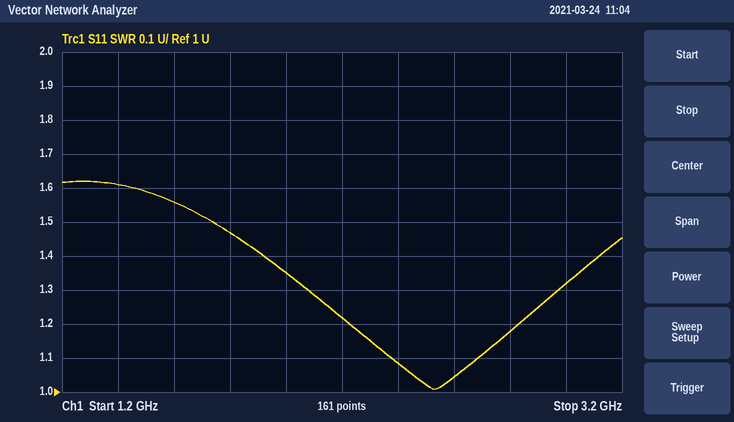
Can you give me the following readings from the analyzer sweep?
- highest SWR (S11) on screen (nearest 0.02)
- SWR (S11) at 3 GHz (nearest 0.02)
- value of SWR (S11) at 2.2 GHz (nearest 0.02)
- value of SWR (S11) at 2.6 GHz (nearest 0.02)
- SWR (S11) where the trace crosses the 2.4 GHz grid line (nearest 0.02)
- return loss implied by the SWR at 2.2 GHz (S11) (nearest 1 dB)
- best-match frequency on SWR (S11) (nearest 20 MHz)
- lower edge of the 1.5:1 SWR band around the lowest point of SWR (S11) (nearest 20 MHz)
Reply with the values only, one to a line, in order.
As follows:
1.62
1.32
1.22
1.04
1.08
20 dB
2.52 GHz
1.74 GHz
